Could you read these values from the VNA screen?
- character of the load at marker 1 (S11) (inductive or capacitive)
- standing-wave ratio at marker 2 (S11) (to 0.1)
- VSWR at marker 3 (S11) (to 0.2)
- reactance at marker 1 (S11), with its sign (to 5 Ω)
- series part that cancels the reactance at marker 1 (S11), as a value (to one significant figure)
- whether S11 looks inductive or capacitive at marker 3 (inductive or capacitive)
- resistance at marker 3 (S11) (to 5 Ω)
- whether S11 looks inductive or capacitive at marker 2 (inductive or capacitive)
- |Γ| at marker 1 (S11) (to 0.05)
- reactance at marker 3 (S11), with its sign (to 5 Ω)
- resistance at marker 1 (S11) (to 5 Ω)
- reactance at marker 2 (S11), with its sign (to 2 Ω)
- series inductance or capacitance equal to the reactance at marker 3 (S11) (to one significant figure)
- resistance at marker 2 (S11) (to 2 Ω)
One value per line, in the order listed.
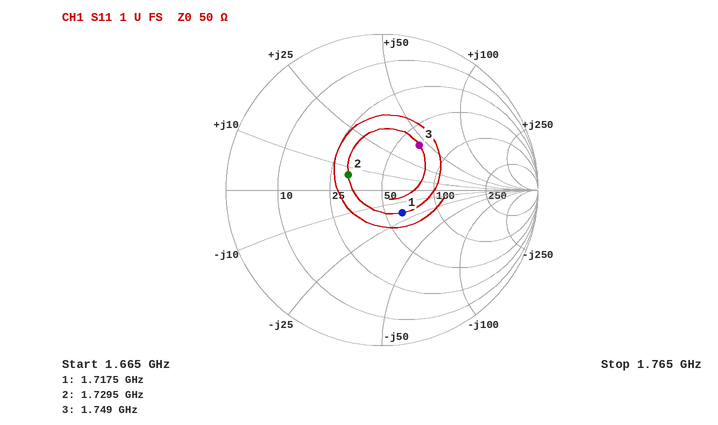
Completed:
capacitive
1.6
2.2
-20 Ω
2 nH
inductive
65 Ω
inductive
0.20
+45 Ω
60 Ω
+6 Ω
4 nH
32 Ω
